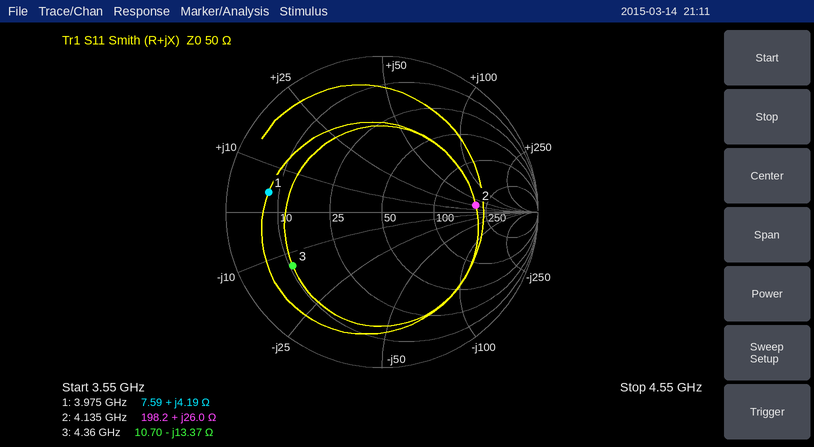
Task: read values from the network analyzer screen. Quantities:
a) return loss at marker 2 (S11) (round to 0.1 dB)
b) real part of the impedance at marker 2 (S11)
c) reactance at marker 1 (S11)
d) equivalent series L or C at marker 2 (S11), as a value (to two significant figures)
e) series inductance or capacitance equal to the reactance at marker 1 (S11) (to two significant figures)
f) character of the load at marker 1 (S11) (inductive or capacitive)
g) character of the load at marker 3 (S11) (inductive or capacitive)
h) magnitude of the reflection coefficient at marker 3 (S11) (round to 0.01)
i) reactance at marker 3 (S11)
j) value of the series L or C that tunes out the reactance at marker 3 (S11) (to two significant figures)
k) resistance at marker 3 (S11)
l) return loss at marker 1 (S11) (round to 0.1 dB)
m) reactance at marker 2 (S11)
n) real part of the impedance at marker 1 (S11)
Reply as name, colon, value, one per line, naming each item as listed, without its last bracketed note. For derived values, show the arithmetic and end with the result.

return loss at marker 2 (S11): 4.4 dB
real part of the impedance at marker 2: 198.2 Ω
reactance at marker 1: +4.19 Ω
equivalent series L or C at marker 2 (S11), as a value: L = 26 Ω/(2π × 4.135 GHz) ≈ 1.00 nH
series inductance or capacitance equal to the reactance at marker 1 (S11): L = 4.19 Ω/(2π × 3.975 GHz) ≈ 168 pH, so 170 pH to two significant figures
character of the load at marker 1 (S11): inductive
character of the load at marker 3 (S11): capacitive
magnitude of the reflection coefficient at marker 3 (S11): 0.67
reactance at marker 3: -13.37 Ω
value of the series L or C that tunes out the reactance at marker 3 (S11): L = 13.37 Ω/(2π × 4.36 GHz) ≈ 488 pH, so 490 pH to two significant figures
resistance at marker 3: 10.70 Ω
return loss at marker 1 (S11): 2.6 dB
reactance at marker 2: +26.0 Ω
real part of the impedance at marker 1: 7.59 Ω
